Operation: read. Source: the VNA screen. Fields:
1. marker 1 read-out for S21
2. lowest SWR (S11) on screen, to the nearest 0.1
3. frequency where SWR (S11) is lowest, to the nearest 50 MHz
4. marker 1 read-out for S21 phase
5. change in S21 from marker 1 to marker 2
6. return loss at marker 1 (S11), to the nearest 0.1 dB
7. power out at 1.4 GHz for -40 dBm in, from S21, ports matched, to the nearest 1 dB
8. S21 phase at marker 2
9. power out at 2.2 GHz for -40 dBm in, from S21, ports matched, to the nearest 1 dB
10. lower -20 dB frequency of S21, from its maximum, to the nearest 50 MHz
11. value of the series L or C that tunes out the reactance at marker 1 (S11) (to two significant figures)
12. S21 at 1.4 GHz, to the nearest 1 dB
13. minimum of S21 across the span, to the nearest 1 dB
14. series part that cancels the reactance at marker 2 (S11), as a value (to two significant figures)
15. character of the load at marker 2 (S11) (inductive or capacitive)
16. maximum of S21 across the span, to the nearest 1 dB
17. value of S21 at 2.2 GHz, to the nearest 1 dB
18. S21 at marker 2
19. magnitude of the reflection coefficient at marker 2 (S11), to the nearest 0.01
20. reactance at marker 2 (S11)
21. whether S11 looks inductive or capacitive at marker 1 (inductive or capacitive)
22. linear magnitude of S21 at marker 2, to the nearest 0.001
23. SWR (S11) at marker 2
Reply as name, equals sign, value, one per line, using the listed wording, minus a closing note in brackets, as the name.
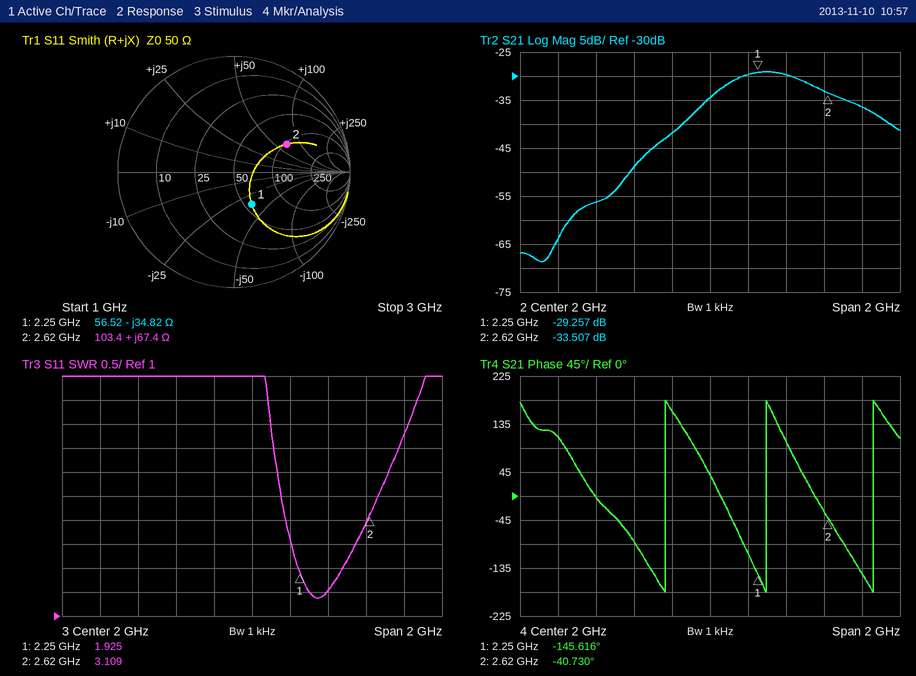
marker 1 read-out for S21 = -29.257 dB
lowest SWR (S11) on screen, to the nearest 0.1 = 1.4
frequency where SWR (S11) is lowest, to the nearest 50 MHz = 2.35 GHz
marker 1 read-out for S21 phase = -145.616°
change in S21 from marker 1 to marker 2 = -4.250 dB
return loss at marker 1 (S11), to the nearest 0.1 dB = 10.0 dB
power out at 1.4 GHz for -40 dBm in, from S21, ports matched, to the nearest 1 dB = -96 dBm
S21 phase at marker 2 = -40.730°
power out at 2.2 GHz for -40 dBm in, from S21, ports matched, to the nearest 1 dB = -70 dBm
lower -20 dB frequency of S21, from its maximum, to the nearest 50 MHz = 1.60 GHz
value of the series L or C that tunes out the reactance at marker 1 (S11) = 2.5 nH
S21 at 1.4 GHz, to the nearest 1 dB = -56 dB
minimum of S21 across the span, to the nearest 1 dB = -69 dB
series part that cancels the reactance at marker 2 (S11), as a value = 900 fF
character of the load at marker 2 (S11) = inductive
maximum of S21 across the span, to the nearest 1 dB = -29 dB
value of S21 at 2.2 GHz, to the nearest 1 dB = -30 dB
S21 at marker 2 = -33.507 dB
magnitude of the reflection coefficient at marker 2 (S11), to the nearest 0.01 = 0.51
reactance at marker 2 = +67.4 Ω
whether S11 looks inductive or capacitive at marker 1 = capacitive
linear magnitude of S21 at marker 2, to the nearest 0.001 = 0.021
SWR (S11) at marker 2 = 3.109
